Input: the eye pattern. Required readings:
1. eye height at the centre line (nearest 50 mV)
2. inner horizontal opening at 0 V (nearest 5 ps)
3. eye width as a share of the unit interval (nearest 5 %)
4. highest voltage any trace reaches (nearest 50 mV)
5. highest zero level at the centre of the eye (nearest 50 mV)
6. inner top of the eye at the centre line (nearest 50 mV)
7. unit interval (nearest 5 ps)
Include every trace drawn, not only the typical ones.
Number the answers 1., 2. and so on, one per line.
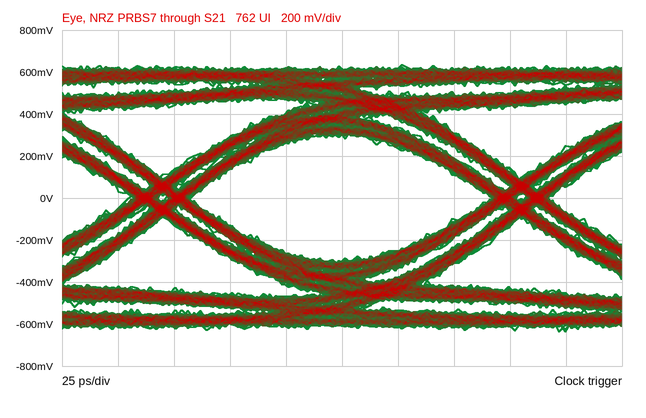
1. 600 mV
2. 135 ps
3. 85 %
4. 650 mV
5. -300 mV
6. 300 mV
7. 160 ps
